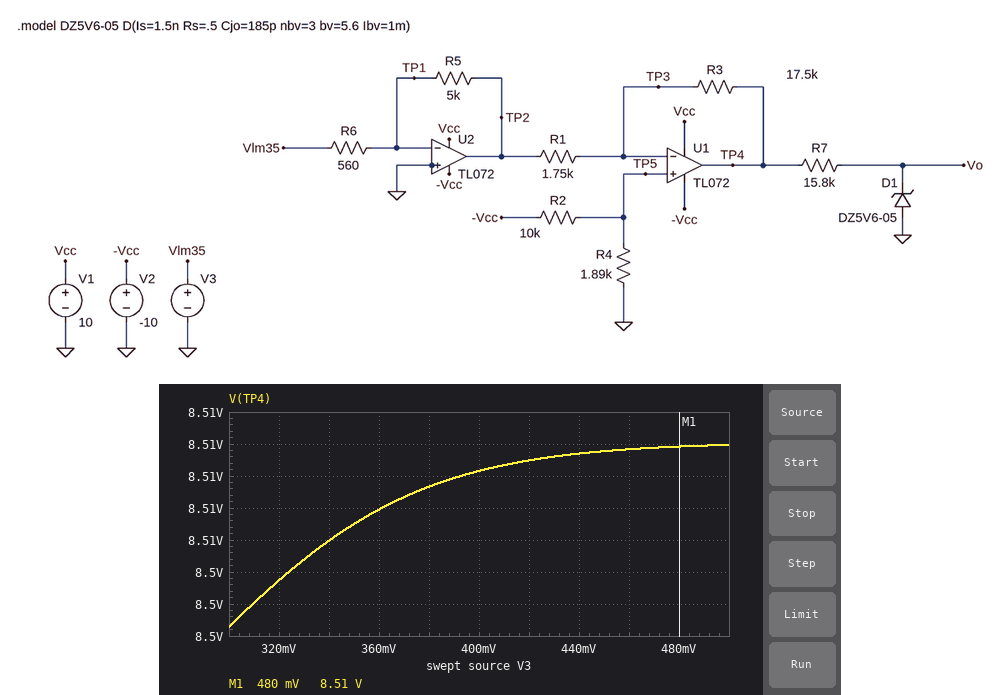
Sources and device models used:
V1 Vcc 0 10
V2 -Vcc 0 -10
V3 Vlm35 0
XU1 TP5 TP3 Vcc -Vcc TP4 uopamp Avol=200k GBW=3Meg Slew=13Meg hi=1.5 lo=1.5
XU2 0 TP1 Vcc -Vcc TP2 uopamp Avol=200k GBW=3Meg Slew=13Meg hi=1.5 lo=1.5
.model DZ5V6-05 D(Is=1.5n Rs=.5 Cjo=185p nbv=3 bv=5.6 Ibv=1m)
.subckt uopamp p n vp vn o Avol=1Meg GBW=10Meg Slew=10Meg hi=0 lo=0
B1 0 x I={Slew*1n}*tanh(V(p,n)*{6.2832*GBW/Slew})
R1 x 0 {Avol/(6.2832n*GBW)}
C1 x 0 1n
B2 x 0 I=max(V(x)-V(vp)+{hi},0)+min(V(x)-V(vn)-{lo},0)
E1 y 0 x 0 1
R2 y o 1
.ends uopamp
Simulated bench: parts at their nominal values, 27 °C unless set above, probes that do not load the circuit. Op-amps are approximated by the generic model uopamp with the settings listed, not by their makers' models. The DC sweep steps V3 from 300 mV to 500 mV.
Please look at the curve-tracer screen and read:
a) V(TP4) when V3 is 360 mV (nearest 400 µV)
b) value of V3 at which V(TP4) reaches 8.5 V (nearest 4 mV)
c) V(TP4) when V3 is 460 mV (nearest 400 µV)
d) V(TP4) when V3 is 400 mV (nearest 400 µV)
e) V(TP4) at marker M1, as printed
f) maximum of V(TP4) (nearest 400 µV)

8.5080 V
324 mV
8.5116 V
8.5104 V
8.51 V
8.5120 V
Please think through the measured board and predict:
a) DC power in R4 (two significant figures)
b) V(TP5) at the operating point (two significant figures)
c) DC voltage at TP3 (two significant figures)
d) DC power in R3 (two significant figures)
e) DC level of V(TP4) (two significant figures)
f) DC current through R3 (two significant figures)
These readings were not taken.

1.3 mW
-1.6 V
-770 mV
3.4 mW
-8.5 V
440 µA
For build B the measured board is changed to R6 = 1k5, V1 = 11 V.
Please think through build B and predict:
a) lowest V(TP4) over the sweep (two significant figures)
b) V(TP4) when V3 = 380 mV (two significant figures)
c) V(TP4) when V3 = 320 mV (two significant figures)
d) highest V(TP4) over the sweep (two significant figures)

-7.5 V
-4.8 V
-6.8 V
-820 mV
